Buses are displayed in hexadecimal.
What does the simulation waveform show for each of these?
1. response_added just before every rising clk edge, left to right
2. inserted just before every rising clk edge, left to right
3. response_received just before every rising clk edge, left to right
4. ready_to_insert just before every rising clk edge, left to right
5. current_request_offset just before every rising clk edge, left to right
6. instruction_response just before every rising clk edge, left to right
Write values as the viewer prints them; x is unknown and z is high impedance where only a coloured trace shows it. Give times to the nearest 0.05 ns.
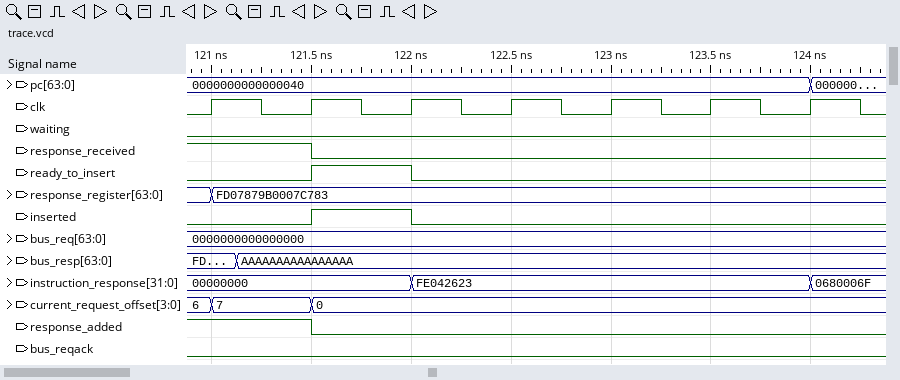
1 1 0 0 0 0 0
0 0 1 0 0 0 0
1 1 0 0 0 0 0
0 0 1 0 0 0 0
6, 7, 0, 0, 0, 0, 0
00000000, 00000000, 00000000, FE042623, FE042623, FE042623, FE042623
